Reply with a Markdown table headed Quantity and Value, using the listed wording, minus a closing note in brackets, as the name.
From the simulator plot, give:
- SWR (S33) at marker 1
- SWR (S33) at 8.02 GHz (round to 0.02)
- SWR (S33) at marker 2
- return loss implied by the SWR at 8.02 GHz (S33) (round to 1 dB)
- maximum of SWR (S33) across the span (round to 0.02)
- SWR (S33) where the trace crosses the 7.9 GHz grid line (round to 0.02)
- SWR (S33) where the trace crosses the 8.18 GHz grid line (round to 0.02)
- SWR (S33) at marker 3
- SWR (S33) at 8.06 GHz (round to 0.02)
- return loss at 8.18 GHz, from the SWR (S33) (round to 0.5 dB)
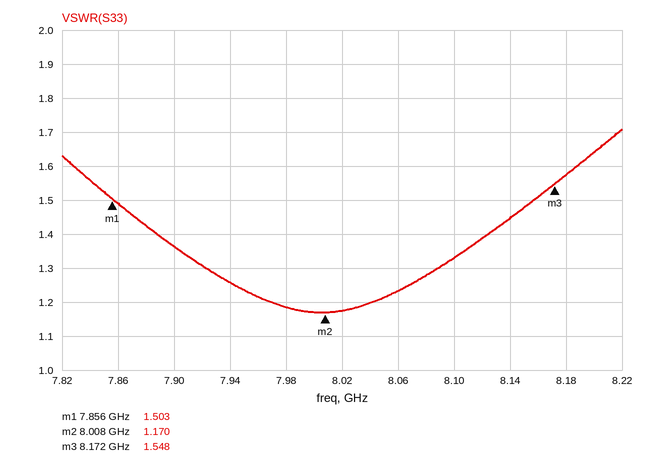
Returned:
| Quantity | Value |
|---|---|
| SWR (S33) at marker 1 | 1.503 |
| SWR (S33) at 8.02 GHz | 1.18 |
| SWR (S33) at marker 2 | 1.170 |
| return loss implied by the SWR at 8.02 GHz (S33) | 22 dB |
| maximum of SWR (S33) across the span | 1.70 |
| SWR (S33) where the trace crosses the 7.9 GHz grid line | 1.36 |
| SWR (S33) where the trace crosses the 8.18 GHz grid line | 1.58 |
| SWR (S33) at marker 3 | 1.548 |
| SWR (S33) at 8.06 GHz | 1.24 |
| return loss at 8.18 GHz, from the SWR (S33) | 13.0 dB |
